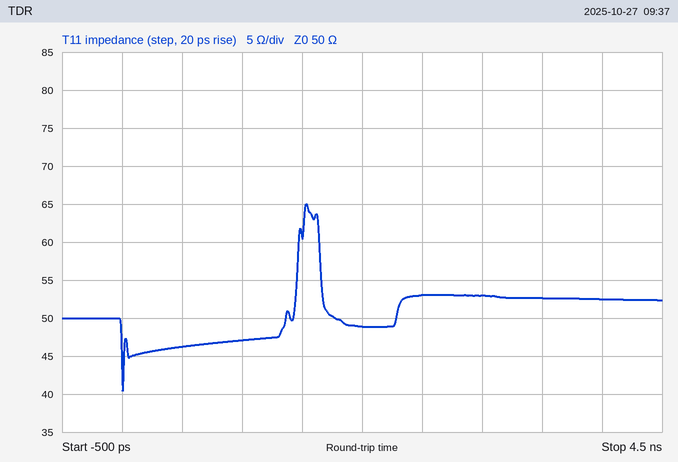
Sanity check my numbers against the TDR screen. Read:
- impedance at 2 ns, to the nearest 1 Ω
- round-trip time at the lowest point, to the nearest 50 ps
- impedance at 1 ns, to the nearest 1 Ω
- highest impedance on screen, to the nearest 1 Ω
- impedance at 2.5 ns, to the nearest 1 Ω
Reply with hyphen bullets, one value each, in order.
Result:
- 49 Ω
- 0 ps
- 47 Ω
- 65 Ω
- 53 Ω
